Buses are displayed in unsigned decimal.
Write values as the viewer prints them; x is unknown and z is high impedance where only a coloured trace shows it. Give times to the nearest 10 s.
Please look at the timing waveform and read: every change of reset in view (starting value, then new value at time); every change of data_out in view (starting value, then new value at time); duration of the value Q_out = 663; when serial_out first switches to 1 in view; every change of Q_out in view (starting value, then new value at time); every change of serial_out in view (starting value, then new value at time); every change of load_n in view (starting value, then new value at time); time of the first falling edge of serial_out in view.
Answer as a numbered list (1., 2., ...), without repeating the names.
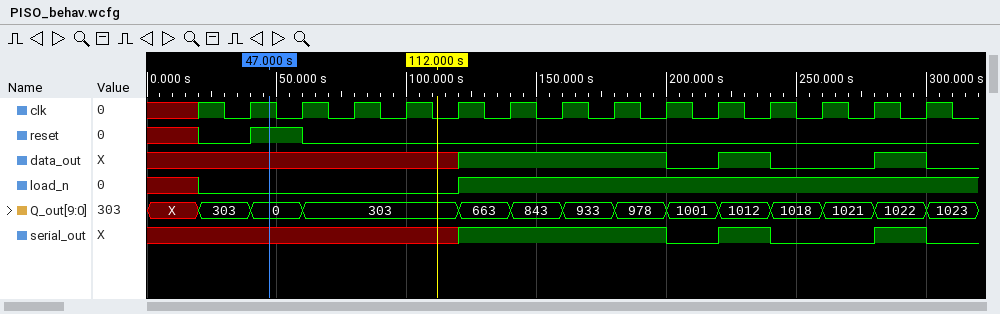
1. x, 0 at 20 s, 1 at 40 s, 0 at 60 s
2. x, 1 at 120 s, 0 at 200 s, 1 at 220 s, 0 at 240 s, 1 at 280 s, 0 at 300 s
3. 20 s
4. 120 s
5. X, 303 at 20 s, 0 at 40 s, 303 at 60 s, 663 at 120 s, 843 at 140 s, 933 at 160 s, 978 at 180 s, 1001 at 200 s, 1012 at 220 s, 1018 at 240 s, 1021 at 260 s, 1022 at 280 s, 1023 at 300 s
6. x, 1 at 120 s, 0 at 200 s, 1 at 220 s, 0 at 240 s, 1 at 280 s, 0 at 300 s
7. x, 0 at 20 s, 1 at 120 s
8. 200 s
